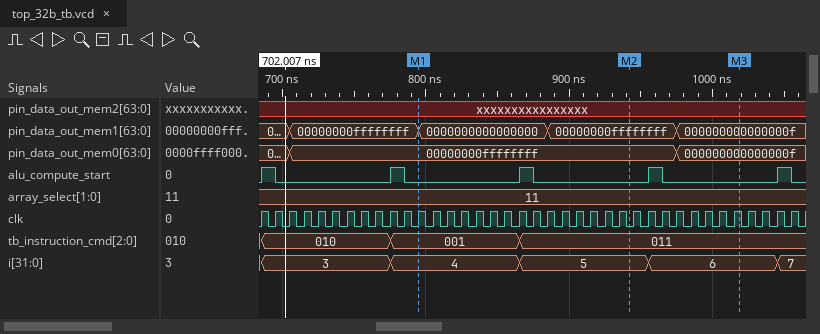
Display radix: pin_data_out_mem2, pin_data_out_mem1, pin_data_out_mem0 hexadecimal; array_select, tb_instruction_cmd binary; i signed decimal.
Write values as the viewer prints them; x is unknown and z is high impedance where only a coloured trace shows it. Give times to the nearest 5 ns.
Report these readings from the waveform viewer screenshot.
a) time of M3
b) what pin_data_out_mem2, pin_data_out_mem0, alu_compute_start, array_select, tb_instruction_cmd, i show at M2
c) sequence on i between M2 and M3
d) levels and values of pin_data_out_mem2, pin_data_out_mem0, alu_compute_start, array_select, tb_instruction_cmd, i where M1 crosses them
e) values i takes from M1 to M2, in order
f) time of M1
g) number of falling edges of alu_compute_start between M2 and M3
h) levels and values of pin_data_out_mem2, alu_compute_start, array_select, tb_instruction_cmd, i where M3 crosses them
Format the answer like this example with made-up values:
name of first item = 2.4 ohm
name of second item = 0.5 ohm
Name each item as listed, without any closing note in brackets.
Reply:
time of M3 = 1020 ns
what pin_data_out_mem2, pin_data_out_mem0, alu_compute_start, array_select, tb_instruction_cmd, i show at M2 = pin_data_out_mem2=xxxxxxxxxxxxxxxx, pin_data_out_mem0=00000000ffffffff, alu_compute_start=0, array_select=11, tb_instruction_cmd=011, i=5
sequence on i between M2 and M3 = 5, 6
levels and values of pin_data_out_mem2, pin_data_out_mem0, alu_compute_start, array_select, tb_instruction_cmd, i where M1 crosses them = pin_data_out_mem2=xxxxxxxxxxxxxxxx, pin_data_out_mem0=00000000ffffffff, alu_compute_start=0, array_select=11, tb_instruction_cmd=001, i=4
values i takes from M1 to M2, in order = 4, 5
time of M1 = 795 ns
number of falling edges of alu_compute_start between M2 and M3 = 1
levels and values of pin_data_out_mem2, alu_compute_start, array_select, tb_instruction_cmd, i where M3 crosses them = pin_data_out_mem2=xxxxxxxxxxxxxxxx, alu_compute_start=0, array_select=11, tb_instruction_cmd=011, i=6
